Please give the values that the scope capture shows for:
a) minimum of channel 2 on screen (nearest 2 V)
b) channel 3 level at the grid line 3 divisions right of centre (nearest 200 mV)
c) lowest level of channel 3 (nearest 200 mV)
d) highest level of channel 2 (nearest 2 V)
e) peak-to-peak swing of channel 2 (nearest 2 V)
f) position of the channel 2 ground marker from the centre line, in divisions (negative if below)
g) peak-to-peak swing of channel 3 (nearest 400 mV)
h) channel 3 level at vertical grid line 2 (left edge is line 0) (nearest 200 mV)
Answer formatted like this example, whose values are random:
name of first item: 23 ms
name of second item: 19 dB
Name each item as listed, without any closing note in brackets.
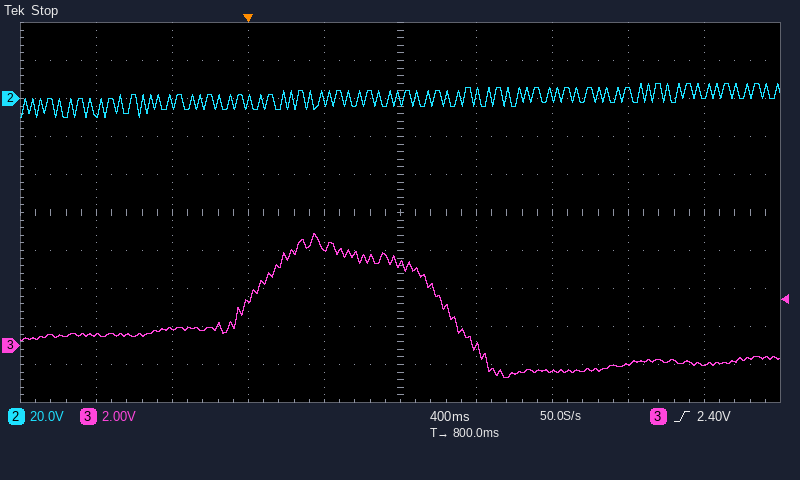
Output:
minimum of channel 2 on screen: -10 V
channel 3 level at the grid line 3 divisions right of centre: -1.0 V
lowest level of channel 3: -1.6 V
highest level of channel 2: 8 V
peak-to-peak swing of channel 2: 18 V
position of the channel 2 ground marker from the centre line, in divisions: +3.0 div
peak-to-peak swing of channel 3: 7.6 V
channel 3 level at vertical grid line 2 (left edge is line 0): 800 mV
